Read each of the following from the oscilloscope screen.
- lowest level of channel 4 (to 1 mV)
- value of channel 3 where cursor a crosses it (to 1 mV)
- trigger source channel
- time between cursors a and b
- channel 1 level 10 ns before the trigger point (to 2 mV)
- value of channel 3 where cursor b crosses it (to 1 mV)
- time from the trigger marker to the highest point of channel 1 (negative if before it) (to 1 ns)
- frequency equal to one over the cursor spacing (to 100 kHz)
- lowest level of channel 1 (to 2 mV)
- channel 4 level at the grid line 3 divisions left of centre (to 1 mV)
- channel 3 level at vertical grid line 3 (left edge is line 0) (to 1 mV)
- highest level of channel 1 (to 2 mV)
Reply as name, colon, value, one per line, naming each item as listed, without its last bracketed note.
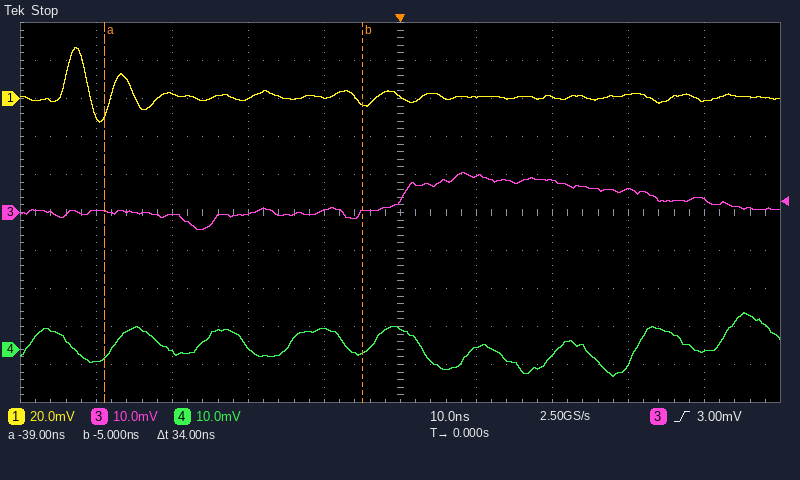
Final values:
lowest level of channel 4: -7 mV
value of channel 3 where cursor a crosses it: 0 mV
trigger source channel: channel 3
time between cursors a and b: 34 ns
channel 1 level 10 ns before the trigger point: 0 mV
value of channel 3 where cursor b crosses it: 0 mV
time from the trigger marker to the highest point of channel 1 (negative if before it): -43 ns
frequency equal to one over the cursor spacing: 29.4 MHz
lowest level of channel 1: -12 mV
channel 4 level at the grid line 3 divisions left of centre: -1 mV
channel 3 level at vertical grid line 3 (left edge is line 0): 0 mV
highest level of channel 1: 26 mV
